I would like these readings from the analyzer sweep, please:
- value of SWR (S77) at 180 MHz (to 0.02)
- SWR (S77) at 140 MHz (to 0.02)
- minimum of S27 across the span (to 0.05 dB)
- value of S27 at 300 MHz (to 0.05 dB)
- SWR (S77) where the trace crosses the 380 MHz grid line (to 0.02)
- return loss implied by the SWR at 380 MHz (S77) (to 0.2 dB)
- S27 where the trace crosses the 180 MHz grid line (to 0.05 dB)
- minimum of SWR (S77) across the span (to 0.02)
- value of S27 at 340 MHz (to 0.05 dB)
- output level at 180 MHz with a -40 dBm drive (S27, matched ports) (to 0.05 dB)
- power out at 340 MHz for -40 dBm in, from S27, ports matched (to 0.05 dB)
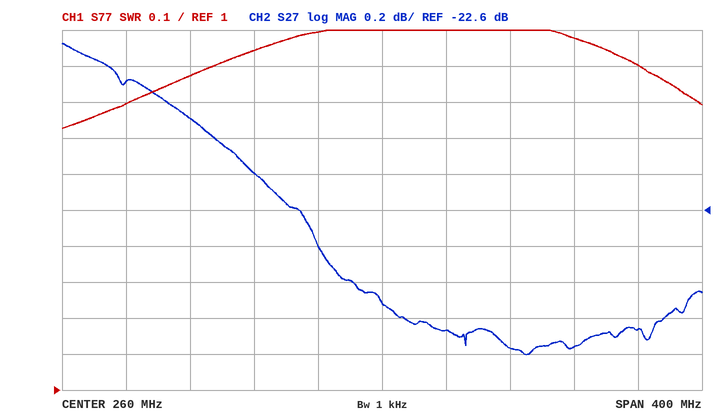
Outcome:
1.94
1.88
-23.40 dB
-23.25 dB
1.98
9.6 dB
-22.40 dB
1.72
-23.35 dB
-62.40 dBm
-63.35 dBm
